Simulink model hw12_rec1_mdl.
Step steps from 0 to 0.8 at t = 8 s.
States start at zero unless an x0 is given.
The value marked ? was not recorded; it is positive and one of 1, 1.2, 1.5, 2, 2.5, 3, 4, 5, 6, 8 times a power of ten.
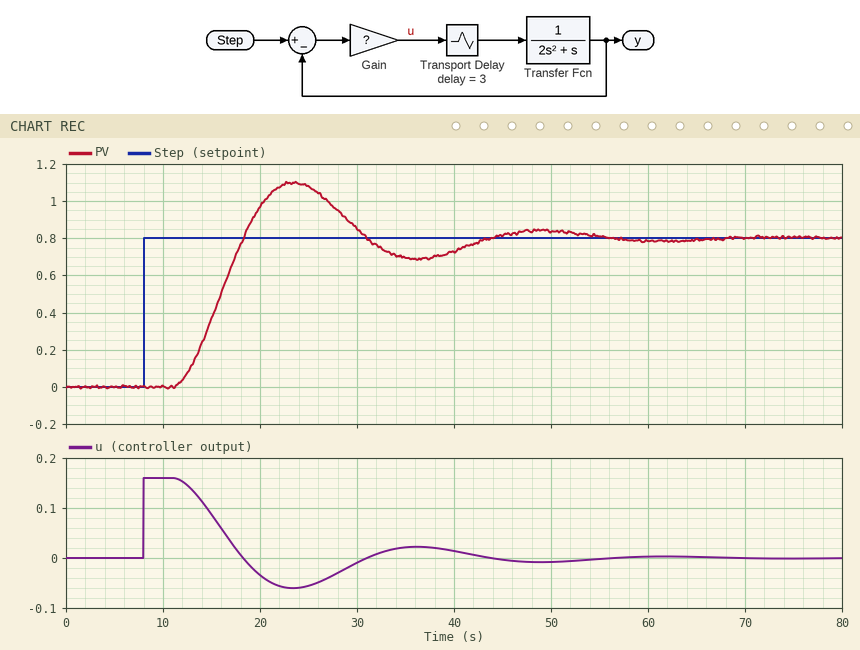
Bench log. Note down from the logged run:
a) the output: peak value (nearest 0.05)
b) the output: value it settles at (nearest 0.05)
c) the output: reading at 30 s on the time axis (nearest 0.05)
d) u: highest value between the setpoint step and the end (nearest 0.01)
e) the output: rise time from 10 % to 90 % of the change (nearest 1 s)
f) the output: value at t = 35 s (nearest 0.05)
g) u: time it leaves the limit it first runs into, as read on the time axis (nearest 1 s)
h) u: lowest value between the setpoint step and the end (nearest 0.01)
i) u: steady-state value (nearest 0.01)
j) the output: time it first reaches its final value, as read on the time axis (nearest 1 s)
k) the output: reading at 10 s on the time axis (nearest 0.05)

1.10
0.80
0.85
0.16
5 s
0.70
12 s
-0.06
0.00
18 s
0.00
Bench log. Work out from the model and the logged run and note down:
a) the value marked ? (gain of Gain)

0.2
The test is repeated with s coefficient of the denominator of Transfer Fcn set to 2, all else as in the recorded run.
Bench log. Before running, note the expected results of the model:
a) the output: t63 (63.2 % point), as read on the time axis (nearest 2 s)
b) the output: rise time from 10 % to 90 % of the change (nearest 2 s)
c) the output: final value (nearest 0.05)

18 s
12 s
0.80
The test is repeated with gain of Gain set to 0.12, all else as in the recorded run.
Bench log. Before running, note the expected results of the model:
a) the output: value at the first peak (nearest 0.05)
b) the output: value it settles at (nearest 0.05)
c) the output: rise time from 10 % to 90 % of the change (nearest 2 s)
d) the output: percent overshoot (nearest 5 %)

0.90
0.80
8 s
10 %
